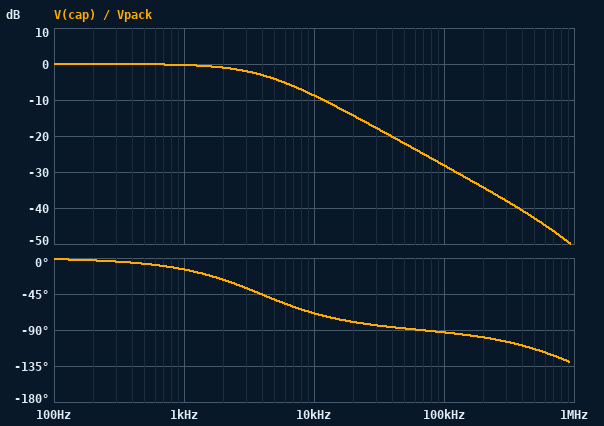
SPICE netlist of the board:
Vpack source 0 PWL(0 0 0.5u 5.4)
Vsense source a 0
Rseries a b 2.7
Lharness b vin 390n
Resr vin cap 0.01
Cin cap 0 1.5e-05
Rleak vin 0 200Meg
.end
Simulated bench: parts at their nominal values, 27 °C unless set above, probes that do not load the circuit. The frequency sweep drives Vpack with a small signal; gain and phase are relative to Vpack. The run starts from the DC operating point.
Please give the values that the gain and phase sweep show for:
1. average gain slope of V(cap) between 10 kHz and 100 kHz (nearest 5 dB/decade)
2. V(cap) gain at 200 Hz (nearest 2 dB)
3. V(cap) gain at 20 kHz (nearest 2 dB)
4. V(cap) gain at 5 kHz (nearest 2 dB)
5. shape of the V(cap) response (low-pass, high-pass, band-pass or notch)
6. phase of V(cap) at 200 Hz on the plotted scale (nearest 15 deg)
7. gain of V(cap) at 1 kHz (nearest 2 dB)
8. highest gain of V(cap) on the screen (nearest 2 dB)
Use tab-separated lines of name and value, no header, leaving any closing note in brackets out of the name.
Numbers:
average gain slope of V(cap) between 10 kHz and 100 kHz	-20 dB/decade
V(cap) gain at 200 Hz	0 dB
V(cap) gain at 20 kHz	-14 dB
V(cap) gain at 5 kHz	-4 dB
shape of the V(cap) response	low-pass
phase of V(cap) at 200 Hz on the plotted scale	0 deg
gain of V(cap) at 1 kHz	0 dB
highest gain of V(cap) on the screen	0 dB
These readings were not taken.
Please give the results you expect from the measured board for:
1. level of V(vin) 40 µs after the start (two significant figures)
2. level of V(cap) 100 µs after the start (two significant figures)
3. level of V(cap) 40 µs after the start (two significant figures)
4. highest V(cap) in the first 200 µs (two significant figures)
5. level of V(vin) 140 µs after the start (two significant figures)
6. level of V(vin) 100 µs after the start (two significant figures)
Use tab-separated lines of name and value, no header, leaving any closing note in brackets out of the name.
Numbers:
level of V(vin) 40 µs after the start	3.4 V
level of V(cap) 100 µs after the start	4.9 V
level of V(cap) 40 µs after the start	3.4 V
highest V(cap) in the first 200 µs	5.4 V
level of V(vin) 140 µs after the start	5.2 V
level of V(vin) 100 µs after the start	4.9 V
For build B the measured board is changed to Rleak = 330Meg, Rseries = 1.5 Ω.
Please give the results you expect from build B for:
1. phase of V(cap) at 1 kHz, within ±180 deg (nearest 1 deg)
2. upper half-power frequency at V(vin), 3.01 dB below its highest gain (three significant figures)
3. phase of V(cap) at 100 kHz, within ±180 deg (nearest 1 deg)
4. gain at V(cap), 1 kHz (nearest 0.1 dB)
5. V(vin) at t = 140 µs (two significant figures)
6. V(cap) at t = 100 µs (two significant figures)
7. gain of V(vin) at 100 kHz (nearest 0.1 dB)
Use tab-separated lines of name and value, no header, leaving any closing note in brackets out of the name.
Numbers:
phase of V(cap) at 1 kHz, within ±180 deg	-8 deg
upper half-power frequency at V(vin), 3.01 dB below its highest gain	7.11 kHz
phase of V(cap) at 100 kHz, within ±180 deg	-95 deg
gain at V(cap), 1 kHz	-0.1 dB
V(vin) at t = 140 µs	5.4 V
V(cap) at t = 100 µs	5.3 V
gain of V(vin) at 100 kHz	-23.1 dB
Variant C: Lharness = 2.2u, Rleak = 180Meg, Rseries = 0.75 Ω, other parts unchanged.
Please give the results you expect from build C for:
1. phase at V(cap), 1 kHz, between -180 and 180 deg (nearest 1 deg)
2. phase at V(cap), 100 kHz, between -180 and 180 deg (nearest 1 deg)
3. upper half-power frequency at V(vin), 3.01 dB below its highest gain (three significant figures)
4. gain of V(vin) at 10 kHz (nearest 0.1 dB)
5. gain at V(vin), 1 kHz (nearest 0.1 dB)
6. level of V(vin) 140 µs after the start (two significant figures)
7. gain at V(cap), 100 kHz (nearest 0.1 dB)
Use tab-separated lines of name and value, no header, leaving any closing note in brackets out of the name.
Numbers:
phase at V(cap), 1 kHz, between -180 and 180 deg	-4 deg
phase at V(cap), 100 kHz, between -180 and 180 deg	-149 deg
upper half-power frequency at V(vin), 3.01 dB below its highest gain	18.0 kHz
gain of V(vin) at 10 kHz	-1.0 dB
gain at V(vin), 1 kHz	0 dB
level of V(vin) 140 µs after the start	5.4 V
gain at V(cap), 100 kHz	-22.9 dB
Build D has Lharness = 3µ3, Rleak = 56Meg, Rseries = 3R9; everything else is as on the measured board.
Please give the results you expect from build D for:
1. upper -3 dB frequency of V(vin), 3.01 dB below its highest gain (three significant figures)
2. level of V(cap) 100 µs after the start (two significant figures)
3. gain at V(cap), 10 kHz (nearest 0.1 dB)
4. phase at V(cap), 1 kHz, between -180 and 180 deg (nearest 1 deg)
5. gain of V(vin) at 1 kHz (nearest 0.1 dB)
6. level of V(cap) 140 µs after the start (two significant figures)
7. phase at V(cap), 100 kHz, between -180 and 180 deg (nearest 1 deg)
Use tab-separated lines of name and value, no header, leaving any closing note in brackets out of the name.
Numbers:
upper -3 dB frequency of V(vin), 3.01 dB below its highest gain	2.75 kHz
level of V(cap) 100 µs after the start	4.4 V
gain at V(cap), 10 kHz	-11.5 dB
phase at V(cap), 1 kHz, between -180 and 180 deg	-20 deg
gain of V(vin) at 1 kHz	-0.5 dB
level of V(cap) 140 µs after the start	4.9 V
phase at V(cap), 100 kHz, between -180 and 180 deg	-117 deg
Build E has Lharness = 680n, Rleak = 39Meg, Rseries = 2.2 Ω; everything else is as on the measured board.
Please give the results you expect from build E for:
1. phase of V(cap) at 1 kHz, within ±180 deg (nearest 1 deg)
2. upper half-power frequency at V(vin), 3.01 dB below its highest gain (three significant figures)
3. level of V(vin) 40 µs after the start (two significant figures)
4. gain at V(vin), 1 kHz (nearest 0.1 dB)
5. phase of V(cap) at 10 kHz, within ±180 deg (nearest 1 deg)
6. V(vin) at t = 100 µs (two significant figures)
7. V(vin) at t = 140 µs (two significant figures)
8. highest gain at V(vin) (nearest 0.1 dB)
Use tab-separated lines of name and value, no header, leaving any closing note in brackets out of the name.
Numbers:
phase of V(cap) at 1 kHz, within ±180 deg	-12 deg
upper half-power frequency at V(vin), 3.01 dB below its highest gain	4.85 kHz
level of V(vin) 40 µs after the start	3.8 V
gain at V(vin), 1 kHz	-0.2 dB
phase of V(cap) at 10 kHz, within ±180 deg	-65 deg
V(vin) at t = 100 µs	5.1 V
V(vin) at t = 140 µs	5.3 V
highest gain at V(vin)	0 dB
